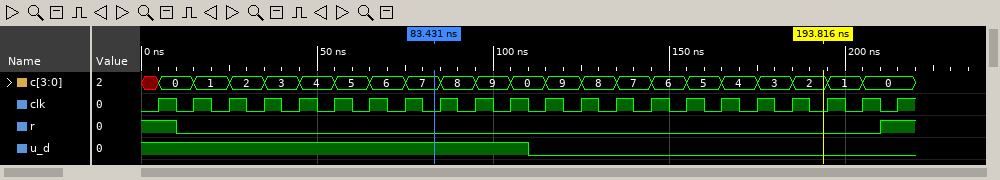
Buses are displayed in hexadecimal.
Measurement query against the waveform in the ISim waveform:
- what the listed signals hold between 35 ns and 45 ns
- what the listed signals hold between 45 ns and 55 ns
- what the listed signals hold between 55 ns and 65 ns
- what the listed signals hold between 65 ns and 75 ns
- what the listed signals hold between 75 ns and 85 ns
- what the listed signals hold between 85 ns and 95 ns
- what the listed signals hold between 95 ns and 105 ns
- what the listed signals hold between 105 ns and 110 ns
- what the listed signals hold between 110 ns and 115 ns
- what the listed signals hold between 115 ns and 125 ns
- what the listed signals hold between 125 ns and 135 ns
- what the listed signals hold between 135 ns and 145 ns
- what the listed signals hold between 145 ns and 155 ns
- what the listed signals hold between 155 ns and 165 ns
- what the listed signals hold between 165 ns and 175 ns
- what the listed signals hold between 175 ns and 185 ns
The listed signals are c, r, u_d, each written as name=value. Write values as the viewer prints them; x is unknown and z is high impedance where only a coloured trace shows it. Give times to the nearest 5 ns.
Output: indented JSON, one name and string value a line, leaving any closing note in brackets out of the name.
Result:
{
  "what the listed signals hold between 35 ns and 45 ns": "c=3, r=0, u_d=1",
  "what the listed signals hold between 45 ns and 55 ns": "c=4, r=0, u_d=1",
  "what the listed signals hold between 55 ns and 65 ns": "c=5, r=0, u_d=1",
  "what the listed signals hold between 65 ns and 75 ns": "c=6, r=0, u_d=1",
  "what the listed signals hold between 75 ns and 85 ns": "c=7, r=0, u_d=1",
  "what the listed signals hold between 85 ns and 95 ns": "c=8, r=0, u_d=1",
  "what the listed signals hold between 95 ns and 105 ns": "c=9, r=0, u_d=1",
  "what the listed signals hold between 105 ns and 110 ns": "c=0, r=0, u_d=1",
  "what the listed signals hold between 110 ns and 115 ns": "c=0, r=0, u_d=0",
  "what the listed signals hold between 115 ns and 125 ns": "c=9, r=0, u_d=0",
  "what the listed signals hold between 125 ns and 135 ns": "c=8, r=0, u_d=0",
  "what the listed signals hold between 135 ns and 145 ns": "c=7, r=0, u_d=0",
  "what the listed signals hold between 145 ns and 155 ns": "c=6, r=0, u_d=0",
  "what the listed signals hold between 155 ns and 165 ns": "c=5, r=0, u_d=0",
  "what the listed signals hold between 165 ns and 175 ns": "c=4, r=0, u_d=0",
  "what the listed signals hold between 175 ns and 185 ns": "c=3, r=0, u_d=0"
}
